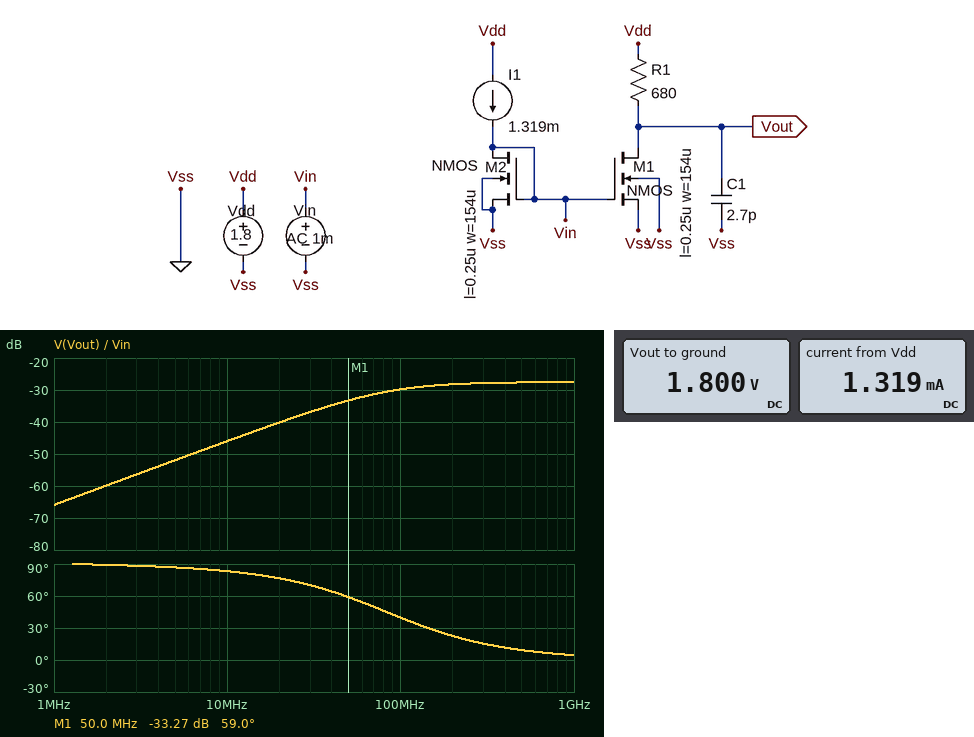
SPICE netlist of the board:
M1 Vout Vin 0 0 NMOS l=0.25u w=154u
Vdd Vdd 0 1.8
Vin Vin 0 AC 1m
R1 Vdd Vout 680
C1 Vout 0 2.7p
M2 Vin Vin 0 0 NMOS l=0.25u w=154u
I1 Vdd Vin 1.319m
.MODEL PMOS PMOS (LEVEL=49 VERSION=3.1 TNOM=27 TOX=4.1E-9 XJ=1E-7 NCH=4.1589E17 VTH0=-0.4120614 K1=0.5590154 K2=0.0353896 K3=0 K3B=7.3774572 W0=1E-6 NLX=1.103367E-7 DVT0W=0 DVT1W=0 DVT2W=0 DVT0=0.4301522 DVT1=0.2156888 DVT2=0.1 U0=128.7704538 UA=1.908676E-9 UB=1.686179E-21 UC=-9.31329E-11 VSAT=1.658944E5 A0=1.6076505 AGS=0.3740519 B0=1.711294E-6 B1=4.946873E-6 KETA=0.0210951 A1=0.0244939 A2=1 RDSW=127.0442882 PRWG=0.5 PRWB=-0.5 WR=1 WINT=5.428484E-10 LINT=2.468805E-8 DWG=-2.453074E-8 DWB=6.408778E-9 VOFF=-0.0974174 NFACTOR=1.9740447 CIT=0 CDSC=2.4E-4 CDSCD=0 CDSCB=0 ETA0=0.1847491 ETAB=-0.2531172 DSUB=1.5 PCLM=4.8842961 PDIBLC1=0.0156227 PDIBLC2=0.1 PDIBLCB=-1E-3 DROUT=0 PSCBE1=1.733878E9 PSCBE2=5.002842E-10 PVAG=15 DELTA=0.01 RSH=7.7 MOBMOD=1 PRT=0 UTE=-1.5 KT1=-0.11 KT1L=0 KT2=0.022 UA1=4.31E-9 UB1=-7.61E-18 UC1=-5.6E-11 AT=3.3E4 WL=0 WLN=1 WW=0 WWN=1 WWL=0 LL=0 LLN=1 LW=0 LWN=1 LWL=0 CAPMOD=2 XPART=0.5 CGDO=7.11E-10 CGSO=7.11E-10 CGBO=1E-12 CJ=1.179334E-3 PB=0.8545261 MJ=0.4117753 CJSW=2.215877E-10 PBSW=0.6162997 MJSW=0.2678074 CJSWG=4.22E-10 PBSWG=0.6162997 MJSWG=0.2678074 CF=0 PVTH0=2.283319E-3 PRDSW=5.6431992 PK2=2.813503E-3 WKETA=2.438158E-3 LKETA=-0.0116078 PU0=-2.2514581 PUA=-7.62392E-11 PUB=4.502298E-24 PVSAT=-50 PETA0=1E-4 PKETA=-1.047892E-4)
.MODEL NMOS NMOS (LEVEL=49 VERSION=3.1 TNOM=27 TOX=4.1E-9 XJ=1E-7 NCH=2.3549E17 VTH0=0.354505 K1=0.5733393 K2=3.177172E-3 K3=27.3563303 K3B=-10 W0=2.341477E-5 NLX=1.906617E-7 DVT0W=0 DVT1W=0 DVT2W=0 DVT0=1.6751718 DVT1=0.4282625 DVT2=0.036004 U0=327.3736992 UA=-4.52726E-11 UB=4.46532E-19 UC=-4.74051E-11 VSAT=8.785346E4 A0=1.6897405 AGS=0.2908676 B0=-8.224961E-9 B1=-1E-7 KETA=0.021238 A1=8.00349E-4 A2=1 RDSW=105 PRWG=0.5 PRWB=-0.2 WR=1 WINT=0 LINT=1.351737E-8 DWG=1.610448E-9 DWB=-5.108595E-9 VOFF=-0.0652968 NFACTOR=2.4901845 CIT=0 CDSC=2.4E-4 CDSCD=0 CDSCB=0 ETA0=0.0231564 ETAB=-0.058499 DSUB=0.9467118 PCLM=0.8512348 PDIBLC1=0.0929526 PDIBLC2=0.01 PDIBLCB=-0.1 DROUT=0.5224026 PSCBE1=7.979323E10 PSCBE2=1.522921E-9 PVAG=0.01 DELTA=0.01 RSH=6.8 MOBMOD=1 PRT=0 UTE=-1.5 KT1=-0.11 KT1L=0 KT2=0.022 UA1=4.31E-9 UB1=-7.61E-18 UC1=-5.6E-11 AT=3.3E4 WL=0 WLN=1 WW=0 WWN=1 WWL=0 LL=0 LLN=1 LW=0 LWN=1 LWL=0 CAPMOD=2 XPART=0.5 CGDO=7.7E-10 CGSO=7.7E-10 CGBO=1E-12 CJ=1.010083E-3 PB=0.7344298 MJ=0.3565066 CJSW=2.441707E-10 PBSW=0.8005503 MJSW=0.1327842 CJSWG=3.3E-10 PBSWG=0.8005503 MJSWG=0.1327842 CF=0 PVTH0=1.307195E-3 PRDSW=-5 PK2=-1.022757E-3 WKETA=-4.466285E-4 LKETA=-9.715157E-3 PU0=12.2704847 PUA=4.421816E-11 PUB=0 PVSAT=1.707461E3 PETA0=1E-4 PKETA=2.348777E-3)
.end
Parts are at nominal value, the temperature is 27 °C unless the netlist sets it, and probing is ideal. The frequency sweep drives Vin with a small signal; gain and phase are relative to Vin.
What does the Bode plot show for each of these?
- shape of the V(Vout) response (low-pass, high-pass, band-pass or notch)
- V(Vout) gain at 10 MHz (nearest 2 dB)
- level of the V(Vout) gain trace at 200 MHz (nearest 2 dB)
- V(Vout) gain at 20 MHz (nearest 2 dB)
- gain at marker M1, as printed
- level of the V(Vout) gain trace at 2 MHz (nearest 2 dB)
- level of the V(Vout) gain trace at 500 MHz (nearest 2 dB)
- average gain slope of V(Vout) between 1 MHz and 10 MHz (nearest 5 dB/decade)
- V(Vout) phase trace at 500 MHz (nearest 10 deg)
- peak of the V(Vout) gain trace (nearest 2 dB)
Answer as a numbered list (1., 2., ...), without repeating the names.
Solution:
1. high-pass
2. -46 dB
3. -28 dB
4. -40 dB
5. -33.27 dB
6. -60 dB
7. -28 dB
8. 20 dB/decade
9. 10 deg
10. -28 dB
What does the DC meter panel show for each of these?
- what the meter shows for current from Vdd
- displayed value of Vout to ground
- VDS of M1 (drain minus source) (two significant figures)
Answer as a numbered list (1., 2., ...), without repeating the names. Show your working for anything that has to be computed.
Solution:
1. 1.319 mA
2. 1.800 V
3. 1.8 V = 1.8 V
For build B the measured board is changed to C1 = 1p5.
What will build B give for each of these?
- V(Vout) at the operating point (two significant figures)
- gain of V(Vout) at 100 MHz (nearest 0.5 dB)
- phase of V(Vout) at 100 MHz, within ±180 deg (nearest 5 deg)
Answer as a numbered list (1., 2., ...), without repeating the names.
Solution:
1. 1.8 V
2. -27.5 dB
3. 55 deg
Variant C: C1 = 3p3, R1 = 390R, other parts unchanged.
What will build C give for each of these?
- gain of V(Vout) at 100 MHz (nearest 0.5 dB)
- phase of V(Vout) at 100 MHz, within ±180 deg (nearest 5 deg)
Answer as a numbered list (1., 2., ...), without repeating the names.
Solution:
1. -33.0 dB
2. 50 deg
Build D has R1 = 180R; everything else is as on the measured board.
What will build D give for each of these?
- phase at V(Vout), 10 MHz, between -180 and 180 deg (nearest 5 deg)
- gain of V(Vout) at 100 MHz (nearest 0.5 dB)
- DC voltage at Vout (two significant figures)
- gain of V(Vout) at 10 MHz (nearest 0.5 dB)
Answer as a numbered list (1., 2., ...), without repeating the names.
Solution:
1. 90 deg
2. -38.0 dB
3. 1.8 V
4. -57.5 dB
